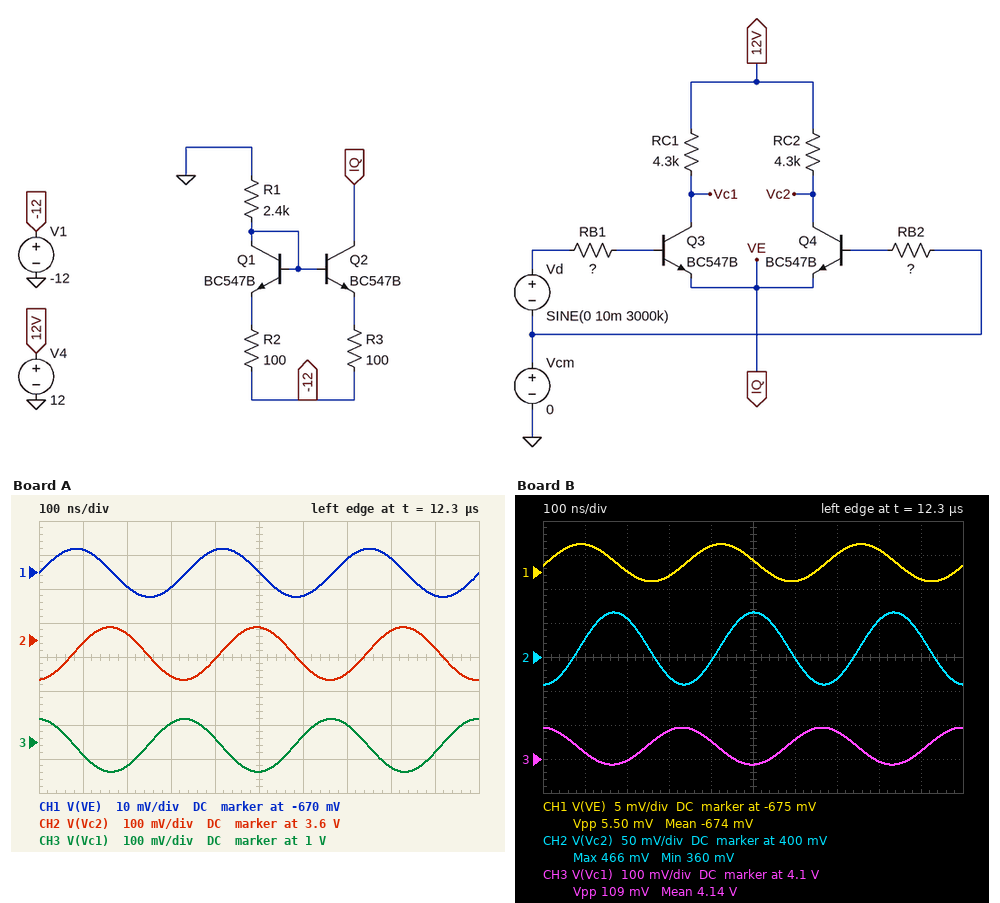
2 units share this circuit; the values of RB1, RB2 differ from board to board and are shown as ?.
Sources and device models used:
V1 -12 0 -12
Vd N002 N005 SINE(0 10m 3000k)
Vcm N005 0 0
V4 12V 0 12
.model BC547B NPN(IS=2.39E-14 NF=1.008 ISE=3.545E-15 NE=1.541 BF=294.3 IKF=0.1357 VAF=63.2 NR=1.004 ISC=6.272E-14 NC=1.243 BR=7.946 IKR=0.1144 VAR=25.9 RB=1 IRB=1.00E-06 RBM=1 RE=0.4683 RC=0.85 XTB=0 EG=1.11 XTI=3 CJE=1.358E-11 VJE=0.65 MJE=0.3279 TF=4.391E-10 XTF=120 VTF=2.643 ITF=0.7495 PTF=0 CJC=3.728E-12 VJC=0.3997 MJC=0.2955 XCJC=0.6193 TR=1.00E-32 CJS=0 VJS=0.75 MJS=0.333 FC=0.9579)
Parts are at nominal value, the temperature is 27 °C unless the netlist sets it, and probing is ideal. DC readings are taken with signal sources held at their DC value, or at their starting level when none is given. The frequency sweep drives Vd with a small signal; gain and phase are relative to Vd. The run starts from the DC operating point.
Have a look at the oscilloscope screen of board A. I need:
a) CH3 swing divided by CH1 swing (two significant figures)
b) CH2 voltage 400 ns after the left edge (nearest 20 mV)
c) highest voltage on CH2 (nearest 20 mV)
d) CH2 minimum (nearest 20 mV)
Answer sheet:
11
3.54 V
3.64 V
3.48 V
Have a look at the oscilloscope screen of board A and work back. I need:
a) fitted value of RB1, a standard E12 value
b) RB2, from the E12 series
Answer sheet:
680 Ω
2.2 kΩ
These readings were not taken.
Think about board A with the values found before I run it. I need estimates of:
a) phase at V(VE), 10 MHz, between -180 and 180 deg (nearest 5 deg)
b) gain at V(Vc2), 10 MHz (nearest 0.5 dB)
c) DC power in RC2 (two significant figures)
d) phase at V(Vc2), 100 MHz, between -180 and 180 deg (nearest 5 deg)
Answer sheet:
-5 deg
7.5 dB
17 mW
-40 deg
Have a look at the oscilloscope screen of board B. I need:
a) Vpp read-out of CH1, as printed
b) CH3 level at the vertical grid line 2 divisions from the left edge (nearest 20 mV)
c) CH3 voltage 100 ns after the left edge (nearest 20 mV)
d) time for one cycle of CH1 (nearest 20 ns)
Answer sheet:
5.50 mV
4.10 V
4.12 V
340 ns
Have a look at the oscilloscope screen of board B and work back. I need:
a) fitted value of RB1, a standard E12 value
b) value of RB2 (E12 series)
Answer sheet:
3.3 kΩ
820 Ω
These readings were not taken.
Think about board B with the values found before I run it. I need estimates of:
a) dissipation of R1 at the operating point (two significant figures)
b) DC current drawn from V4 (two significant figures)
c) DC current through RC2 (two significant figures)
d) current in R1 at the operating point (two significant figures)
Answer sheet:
49 mW
4.5 mA
2.7 mA
4.5 mA
